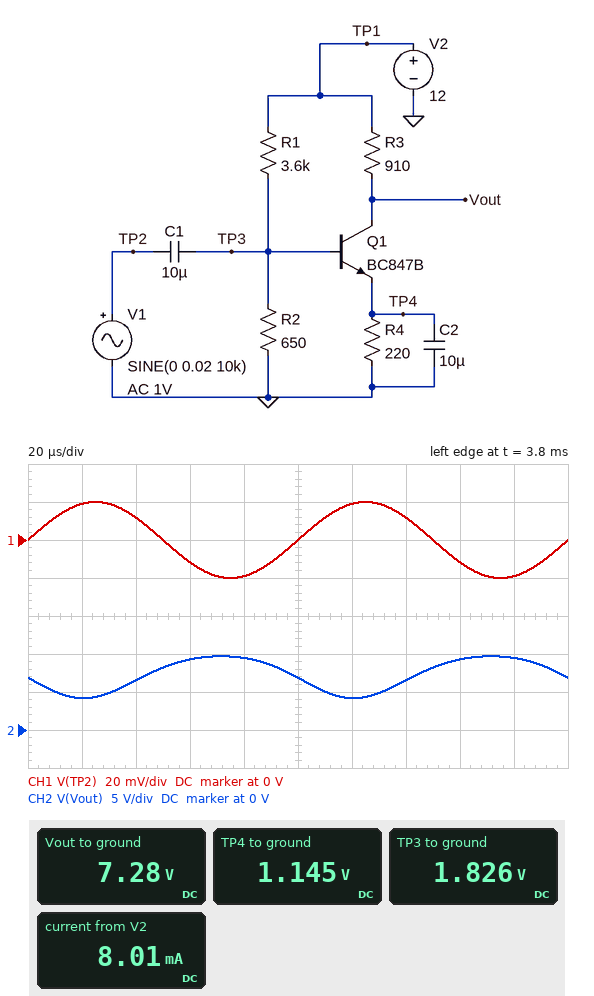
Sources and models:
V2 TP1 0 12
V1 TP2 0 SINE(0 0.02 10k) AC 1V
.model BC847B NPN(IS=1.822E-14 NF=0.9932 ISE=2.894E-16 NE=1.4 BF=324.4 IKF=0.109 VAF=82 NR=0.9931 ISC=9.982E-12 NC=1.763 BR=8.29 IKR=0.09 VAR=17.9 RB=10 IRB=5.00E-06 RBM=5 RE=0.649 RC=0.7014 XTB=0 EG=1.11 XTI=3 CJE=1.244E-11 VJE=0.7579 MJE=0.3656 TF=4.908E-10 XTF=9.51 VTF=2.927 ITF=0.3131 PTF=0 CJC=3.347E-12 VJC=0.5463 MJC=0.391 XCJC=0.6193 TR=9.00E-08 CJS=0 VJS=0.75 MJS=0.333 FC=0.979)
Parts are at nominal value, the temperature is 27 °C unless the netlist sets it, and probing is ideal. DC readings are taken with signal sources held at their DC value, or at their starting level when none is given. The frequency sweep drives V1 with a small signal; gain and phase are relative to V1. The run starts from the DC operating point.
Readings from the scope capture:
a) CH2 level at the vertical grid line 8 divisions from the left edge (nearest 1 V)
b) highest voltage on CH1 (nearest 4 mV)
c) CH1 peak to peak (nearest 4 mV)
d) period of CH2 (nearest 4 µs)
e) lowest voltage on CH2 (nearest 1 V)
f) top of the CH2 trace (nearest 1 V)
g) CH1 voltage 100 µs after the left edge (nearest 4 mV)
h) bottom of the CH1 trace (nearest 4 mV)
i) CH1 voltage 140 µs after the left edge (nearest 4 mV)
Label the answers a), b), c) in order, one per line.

a) 9 V
b) 20 mV
c) 40 mV
d) 100 µs
e) 4 V
f) 10 V
g) 0 V
h) -20 mV
i) 12 mV
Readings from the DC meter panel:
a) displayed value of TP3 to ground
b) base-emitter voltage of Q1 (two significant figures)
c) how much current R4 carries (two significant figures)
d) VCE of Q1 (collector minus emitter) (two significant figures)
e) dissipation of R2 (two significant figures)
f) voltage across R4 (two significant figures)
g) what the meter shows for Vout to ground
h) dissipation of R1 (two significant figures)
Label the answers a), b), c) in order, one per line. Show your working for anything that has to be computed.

a) 1.826 V
b) 1.826 V - 1.145 V = 680 mV
c) (1.145 V) / 220 Ω = 5.2 mA
d) 7.28 V - 1.145 V = 6.1 V
e) (1.826 V)^2 / 650 Ω = 5.1 mW
f) 1.145 V = 1.1 V
g) 7.28 V
h) (12 V - 1.826 V)^2 / 3.6 kΩ = 29 mW
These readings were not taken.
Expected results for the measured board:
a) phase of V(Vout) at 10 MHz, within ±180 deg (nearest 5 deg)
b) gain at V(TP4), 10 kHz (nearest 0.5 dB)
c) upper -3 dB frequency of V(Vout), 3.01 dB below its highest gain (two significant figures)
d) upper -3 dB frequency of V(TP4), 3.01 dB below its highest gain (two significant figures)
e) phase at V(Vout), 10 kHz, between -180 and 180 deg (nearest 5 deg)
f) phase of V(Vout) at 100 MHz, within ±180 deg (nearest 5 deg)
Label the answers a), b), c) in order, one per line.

a) 170 deg
b) -12.0 dB
c) 67 MHz
d) 2.7 kHz
e) -165 deg
f) 110 deg
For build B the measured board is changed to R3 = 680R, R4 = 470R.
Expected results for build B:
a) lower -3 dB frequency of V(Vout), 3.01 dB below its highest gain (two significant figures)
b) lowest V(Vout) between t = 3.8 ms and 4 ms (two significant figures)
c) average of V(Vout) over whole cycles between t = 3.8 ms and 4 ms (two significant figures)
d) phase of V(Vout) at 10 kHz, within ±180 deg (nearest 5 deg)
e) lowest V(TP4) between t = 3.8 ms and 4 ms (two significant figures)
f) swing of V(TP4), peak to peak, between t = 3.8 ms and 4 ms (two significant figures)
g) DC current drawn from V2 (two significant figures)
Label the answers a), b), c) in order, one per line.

a) 1.4 kHz
b) 9.0 V
c) 10 V
d) -170 deg
e) 1.2 V
f) 5.3 mV
g) 5.3 mA
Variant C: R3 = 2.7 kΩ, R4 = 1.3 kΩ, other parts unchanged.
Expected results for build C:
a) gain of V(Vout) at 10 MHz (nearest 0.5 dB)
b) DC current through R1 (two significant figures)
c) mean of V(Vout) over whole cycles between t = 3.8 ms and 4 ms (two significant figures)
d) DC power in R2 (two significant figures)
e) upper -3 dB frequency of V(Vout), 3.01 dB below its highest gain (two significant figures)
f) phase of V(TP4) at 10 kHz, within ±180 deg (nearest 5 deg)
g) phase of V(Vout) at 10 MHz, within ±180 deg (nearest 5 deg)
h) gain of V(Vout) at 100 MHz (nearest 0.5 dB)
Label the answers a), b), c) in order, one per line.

a) 39.0 dB
b) 2.8 mA
c) 9.5 V
d) 5.2 mW
e) 44 MHz
f) -85 deg
g) 165 deg
h) 31.0 dB
